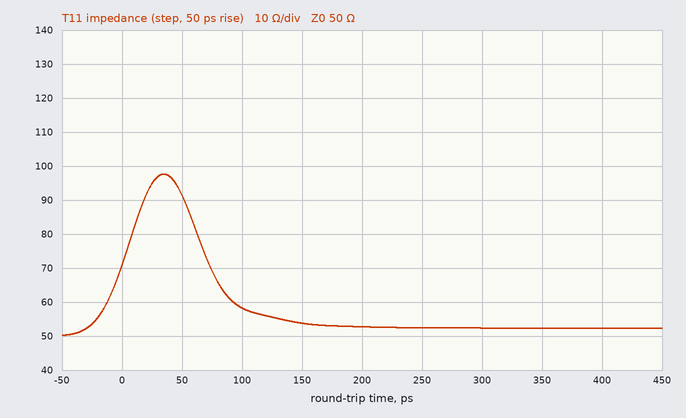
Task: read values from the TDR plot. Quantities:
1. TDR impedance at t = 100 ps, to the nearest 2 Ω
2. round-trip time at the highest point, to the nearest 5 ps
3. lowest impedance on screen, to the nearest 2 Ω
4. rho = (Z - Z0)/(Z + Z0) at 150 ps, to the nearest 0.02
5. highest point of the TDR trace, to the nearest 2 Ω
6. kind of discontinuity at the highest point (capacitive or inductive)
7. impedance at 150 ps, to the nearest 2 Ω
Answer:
58 Ω
35 ps
50 Ω
+0.04
98 Ω
inductive
54 Ω
